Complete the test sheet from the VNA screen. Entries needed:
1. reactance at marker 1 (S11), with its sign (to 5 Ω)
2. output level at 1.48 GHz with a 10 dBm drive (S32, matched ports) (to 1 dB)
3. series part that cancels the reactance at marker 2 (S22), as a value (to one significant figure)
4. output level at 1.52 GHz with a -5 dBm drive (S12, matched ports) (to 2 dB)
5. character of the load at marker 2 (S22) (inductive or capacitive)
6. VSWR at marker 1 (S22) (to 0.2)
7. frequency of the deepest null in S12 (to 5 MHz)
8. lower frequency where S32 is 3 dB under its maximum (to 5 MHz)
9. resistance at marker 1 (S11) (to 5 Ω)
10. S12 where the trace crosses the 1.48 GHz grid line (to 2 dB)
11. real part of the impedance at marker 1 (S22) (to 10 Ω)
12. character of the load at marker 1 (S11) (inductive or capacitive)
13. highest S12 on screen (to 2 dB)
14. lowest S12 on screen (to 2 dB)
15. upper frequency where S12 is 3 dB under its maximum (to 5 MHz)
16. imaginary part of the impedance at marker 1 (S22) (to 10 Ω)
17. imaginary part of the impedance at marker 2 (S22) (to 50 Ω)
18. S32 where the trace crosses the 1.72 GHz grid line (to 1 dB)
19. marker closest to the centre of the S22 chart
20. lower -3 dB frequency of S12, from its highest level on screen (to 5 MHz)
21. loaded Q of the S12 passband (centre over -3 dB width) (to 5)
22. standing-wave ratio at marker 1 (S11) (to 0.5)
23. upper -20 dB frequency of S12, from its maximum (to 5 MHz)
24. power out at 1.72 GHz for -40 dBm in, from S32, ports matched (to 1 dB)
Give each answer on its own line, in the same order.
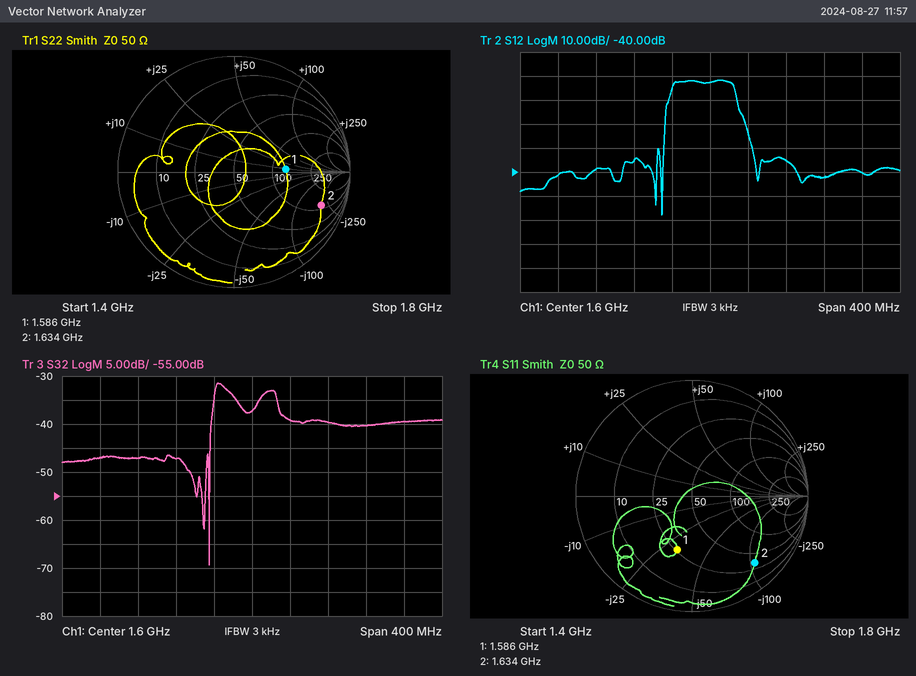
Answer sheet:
-30 Ω
-37 dBm
20 nH
-40 dBm
capacitive
2.6
1.550 GHz
1.560 GHz
25 Ω
-38 dB
130 Ω
capacitive
-2 dB
-58 dB
1.625 GHz
+10 Ω
-200 Ω
-40 dB
marker 1
1.560 GHz
25
3.0
1.640 GHz
-80 dBm
